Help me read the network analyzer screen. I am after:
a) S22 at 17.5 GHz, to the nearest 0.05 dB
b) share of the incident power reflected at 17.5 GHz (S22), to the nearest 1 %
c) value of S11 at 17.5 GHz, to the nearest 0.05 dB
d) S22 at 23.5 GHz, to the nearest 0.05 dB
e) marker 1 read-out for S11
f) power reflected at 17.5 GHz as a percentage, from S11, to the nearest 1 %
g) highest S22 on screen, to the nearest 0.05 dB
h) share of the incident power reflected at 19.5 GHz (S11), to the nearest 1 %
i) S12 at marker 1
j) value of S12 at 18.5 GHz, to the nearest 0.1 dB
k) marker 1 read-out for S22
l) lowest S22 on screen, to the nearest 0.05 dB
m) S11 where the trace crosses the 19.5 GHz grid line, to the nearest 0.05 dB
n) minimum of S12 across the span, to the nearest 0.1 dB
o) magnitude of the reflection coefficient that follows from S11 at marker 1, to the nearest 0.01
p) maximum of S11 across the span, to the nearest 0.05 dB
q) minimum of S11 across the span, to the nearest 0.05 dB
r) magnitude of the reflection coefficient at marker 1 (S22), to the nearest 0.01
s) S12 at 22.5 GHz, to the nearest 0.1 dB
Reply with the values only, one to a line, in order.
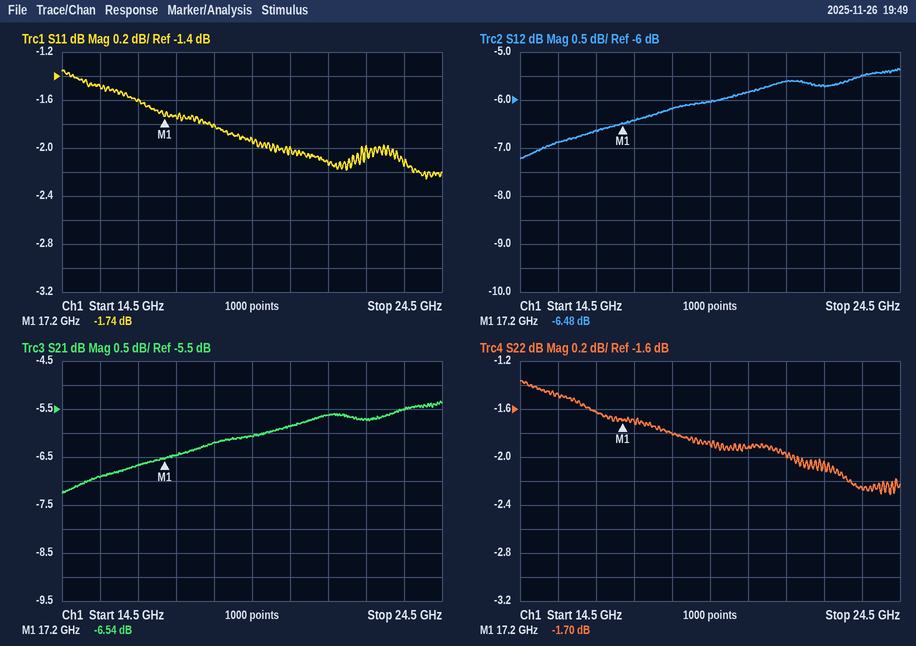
-1.70 dB
68 %
-1.75 dB
-2.25 dB
-1.74 dB
67 %
-1.35 dB
64 %
-6.48 dB
-6.2 dB
-1.70 dB
-2.30 dB
-1.95 dB
-7.2 dB
0.82
-1.35 dB
-2.25 dB
0.82
-5.7 dB
